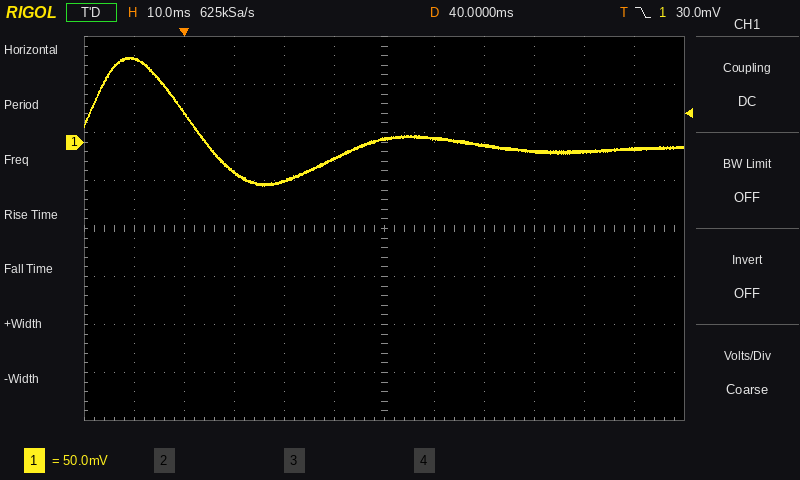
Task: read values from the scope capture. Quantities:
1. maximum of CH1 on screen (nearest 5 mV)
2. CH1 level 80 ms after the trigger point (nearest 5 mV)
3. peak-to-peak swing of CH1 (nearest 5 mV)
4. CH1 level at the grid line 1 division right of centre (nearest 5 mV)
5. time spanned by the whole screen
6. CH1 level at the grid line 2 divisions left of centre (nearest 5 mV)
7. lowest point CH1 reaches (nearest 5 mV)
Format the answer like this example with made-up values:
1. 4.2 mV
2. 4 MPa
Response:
1. 90 mV
2. -10 mV
3. 135 mV
4. 5 mV
5. 120 ms
6. -40 mV
7. -45 mV
